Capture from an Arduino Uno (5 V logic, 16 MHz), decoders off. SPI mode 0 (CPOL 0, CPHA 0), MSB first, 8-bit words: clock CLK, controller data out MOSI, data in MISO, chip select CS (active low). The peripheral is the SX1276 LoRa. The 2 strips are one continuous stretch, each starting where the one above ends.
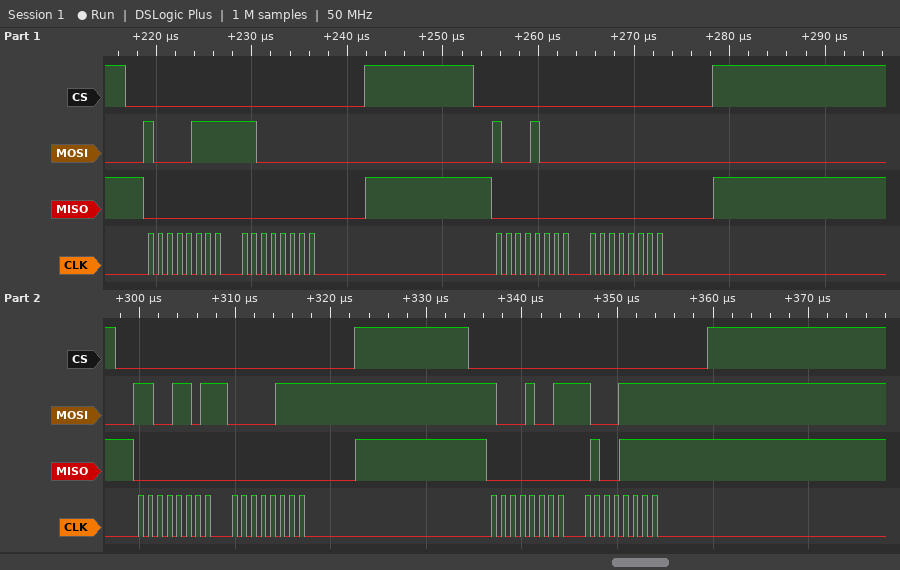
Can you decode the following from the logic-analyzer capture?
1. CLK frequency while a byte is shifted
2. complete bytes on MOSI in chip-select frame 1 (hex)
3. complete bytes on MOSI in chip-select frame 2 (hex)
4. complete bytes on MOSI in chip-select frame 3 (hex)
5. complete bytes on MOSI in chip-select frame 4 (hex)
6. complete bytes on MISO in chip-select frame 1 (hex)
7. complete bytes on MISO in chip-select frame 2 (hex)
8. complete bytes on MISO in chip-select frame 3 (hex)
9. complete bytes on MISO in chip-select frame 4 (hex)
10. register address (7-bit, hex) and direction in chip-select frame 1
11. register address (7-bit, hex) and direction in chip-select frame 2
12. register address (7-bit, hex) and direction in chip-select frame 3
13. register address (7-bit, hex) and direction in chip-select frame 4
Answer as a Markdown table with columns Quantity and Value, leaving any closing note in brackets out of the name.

| Quantity | Value |
|---|---|
| CLK frequency while a byte is shifted | 1 MHz |
| complete bytes on MOSI in chip-select frame 1 | 87 C0 |
| complete bytes on MOSI in chip-select frame 2 | 88 00 |
| complete bytes on MOSI in chip-select frame 3 | CD 07 |
| complete bytes on MOSI in chip-select frame 4 | 89 8F |
| complete bytes on MISO in chip-select frame 1 | 00 00 |
| complete bytes on MISO in chip-select frame 2 | 00 00 |
| complete bytes on MISO in chip-select frame 3 | 00 00 |
| complete bytes on MISO in chip-select frame 4 | 00 4F |
| register address (7-bit, hex) and direction in chip-select frame 1 | 0x07 write |
| register address (7-bit, hex) and direction in chip-select frame 2 | 0x08 write |
| register address (7-bit, hex) and direction in chip-select frame 3 | 0x4D write |
| register address (7-bit, hex) and direction in chip-select frame 4 | 0x09 write |
